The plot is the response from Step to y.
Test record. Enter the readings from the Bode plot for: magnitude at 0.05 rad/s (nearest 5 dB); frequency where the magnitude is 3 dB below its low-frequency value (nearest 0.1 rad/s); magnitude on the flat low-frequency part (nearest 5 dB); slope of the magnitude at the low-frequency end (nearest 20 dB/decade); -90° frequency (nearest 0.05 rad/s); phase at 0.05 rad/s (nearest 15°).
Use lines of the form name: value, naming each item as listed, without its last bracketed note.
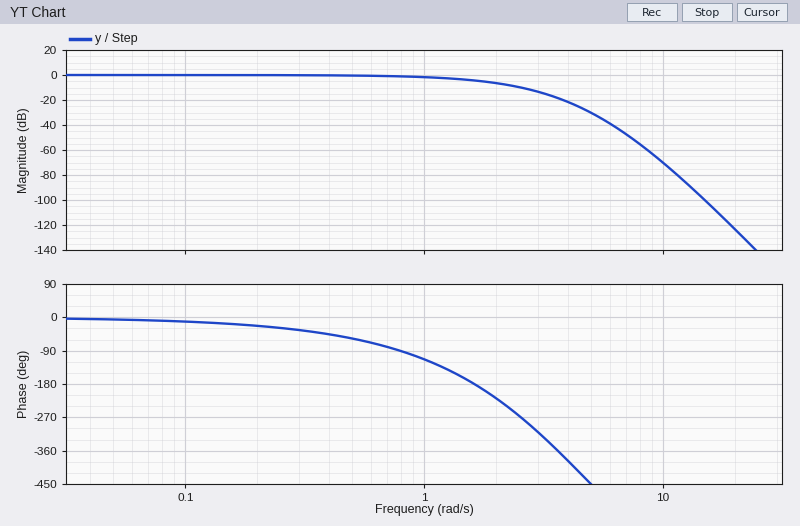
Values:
magnitude at 0.05 rad/s: 0 dB
frequency where the magnitude is 3 dB below its low-frequency value: 1.3 rad/s
magnitude on the flat low-frequency part: 0 dB
slope of the magnitude at the low-frequency end: 0 dB/decade
-90° frequency: 0.80 rad/s
phase at 0.05 rad/s: 0°
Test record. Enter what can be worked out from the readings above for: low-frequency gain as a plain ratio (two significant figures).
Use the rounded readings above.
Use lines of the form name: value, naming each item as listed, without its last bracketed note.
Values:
low-frequency gain as a plain ratio: 1.0
